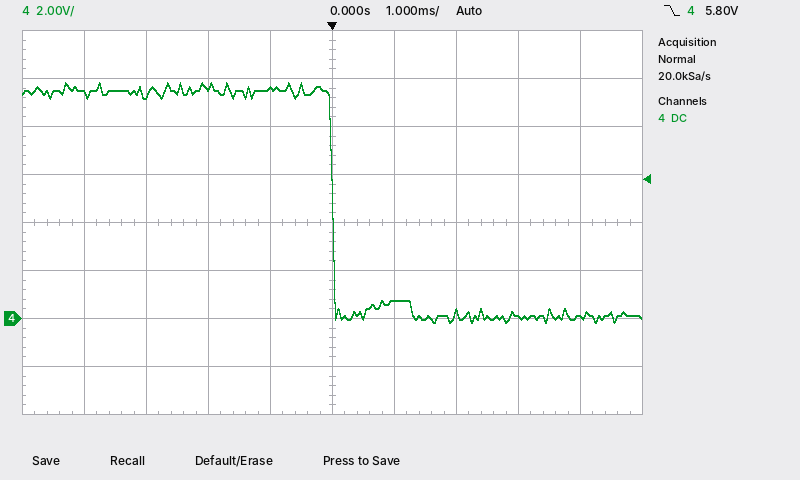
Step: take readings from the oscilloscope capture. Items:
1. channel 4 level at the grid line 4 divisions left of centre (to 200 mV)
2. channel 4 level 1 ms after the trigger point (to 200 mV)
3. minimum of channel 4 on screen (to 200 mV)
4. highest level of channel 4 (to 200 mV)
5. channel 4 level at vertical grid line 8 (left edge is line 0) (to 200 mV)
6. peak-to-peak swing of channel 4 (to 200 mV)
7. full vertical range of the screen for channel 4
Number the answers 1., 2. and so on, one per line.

1. 9.4 V
2. 800 mV
3. -200 mV
4. 9.8 V
5. 0.0 V
6. 10.0 V
7. 16 V
